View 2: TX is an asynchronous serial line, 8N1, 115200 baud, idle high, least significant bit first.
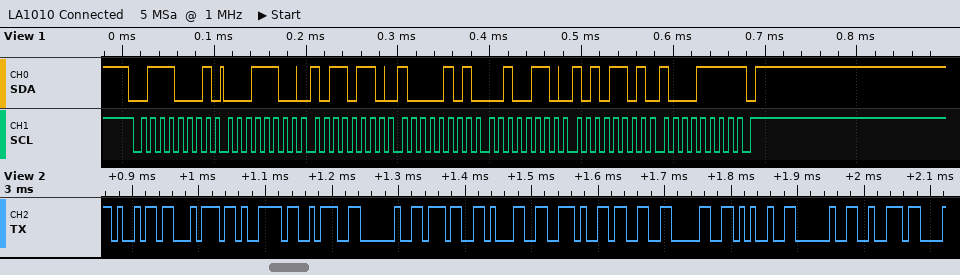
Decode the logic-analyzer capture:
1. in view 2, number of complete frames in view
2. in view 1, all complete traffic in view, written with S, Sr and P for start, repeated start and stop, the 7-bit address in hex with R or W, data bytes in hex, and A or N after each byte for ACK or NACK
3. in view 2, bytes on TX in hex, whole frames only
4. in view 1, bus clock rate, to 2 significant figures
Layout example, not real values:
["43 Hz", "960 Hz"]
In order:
["13", "S 38R A 1C A B6 A 85 A 26 A AD A 8F N P", "0x69 0x74 0x79 0x3A 0x20 0x37 0x31 0x2E 0x33 0x30 0x25 0x20 0x72", "100 kHz"]
